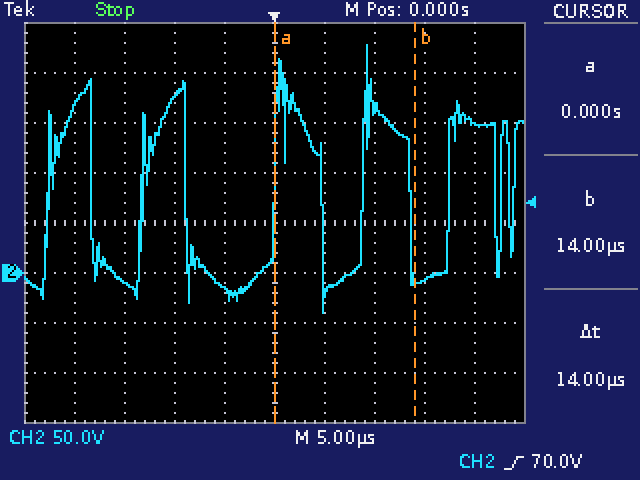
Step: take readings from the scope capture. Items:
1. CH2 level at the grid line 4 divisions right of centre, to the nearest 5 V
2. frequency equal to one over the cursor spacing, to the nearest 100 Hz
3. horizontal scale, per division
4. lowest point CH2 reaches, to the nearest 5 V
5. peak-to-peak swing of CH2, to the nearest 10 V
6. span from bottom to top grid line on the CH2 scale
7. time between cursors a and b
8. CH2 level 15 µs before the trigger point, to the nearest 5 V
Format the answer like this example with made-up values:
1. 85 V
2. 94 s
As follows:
1. 150 V
2. 71.4 kHz
3. 5 µs
4. -40 V
5. 270 V
6. 400 V
7. 14 µs
8. -10 V
